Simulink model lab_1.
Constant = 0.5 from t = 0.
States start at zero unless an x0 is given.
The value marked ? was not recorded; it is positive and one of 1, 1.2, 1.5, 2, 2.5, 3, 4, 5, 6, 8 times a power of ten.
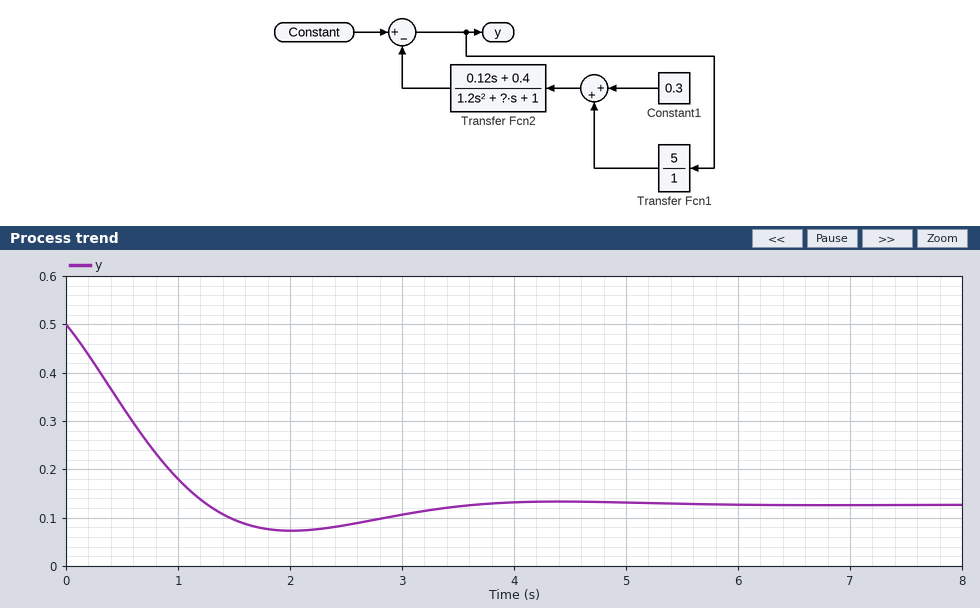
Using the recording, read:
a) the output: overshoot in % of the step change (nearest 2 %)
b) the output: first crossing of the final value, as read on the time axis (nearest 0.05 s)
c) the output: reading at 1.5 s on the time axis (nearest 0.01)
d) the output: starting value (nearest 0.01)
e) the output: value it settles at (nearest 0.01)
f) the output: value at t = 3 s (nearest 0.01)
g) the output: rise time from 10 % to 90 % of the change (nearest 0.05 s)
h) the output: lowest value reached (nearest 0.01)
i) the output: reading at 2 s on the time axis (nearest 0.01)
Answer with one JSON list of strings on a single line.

["14 %", "1.25 s", "0.10", "0.50", "0.13", "0.11", "0.95 s", "0.07", "0.07"]
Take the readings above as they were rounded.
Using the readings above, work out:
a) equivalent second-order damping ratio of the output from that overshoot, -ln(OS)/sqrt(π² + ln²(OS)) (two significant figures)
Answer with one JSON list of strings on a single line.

["0.53"]
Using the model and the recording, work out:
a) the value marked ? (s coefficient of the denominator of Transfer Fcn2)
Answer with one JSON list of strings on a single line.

["1.5"]
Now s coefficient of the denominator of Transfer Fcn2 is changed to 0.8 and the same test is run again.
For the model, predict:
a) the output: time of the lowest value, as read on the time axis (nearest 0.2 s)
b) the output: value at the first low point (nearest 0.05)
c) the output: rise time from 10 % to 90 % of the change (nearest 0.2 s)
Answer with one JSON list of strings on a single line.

["1.8 s", "0.00", "0.8 s"]
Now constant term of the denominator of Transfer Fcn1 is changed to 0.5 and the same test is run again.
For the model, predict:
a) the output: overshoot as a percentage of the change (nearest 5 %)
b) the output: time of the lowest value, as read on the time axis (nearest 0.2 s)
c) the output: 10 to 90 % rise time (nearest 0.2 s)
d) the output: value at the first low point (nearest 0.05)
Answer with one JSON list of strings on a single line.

["15 %", "1.4 s", "0.6 s", "0.00"]
